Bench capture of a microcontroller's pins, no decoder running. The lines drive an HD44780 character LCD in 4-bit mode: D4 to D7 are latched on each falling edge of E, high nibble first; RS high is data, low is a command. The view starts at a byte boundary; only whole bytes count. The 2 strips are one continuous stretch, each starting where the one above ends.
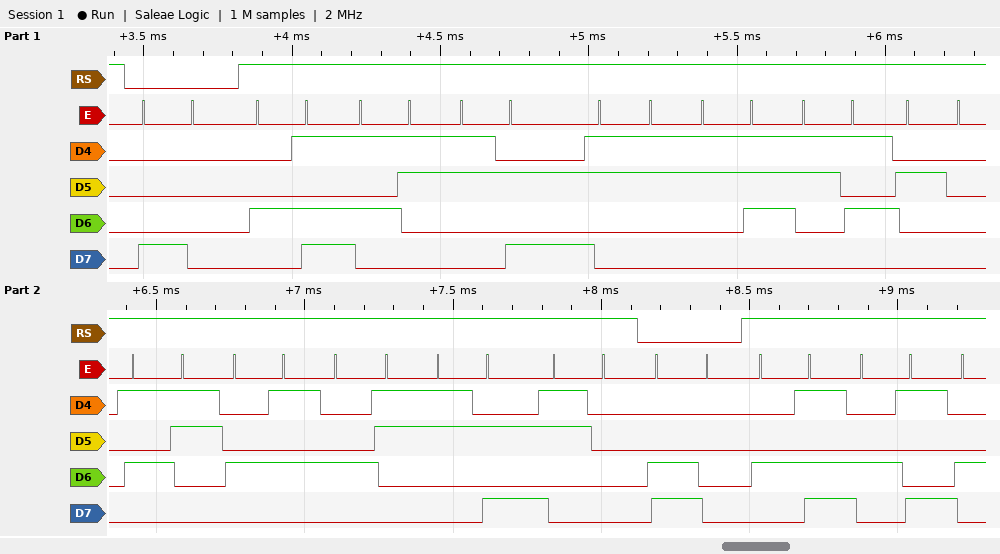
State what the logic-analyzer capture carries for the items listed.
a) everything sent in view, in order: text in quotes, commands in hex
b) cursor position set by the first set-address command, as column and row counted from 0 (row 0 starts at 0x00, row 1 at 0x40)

0x80 "MS:375 SEC:0" 0xC0 "MI"
column 0, row 0
